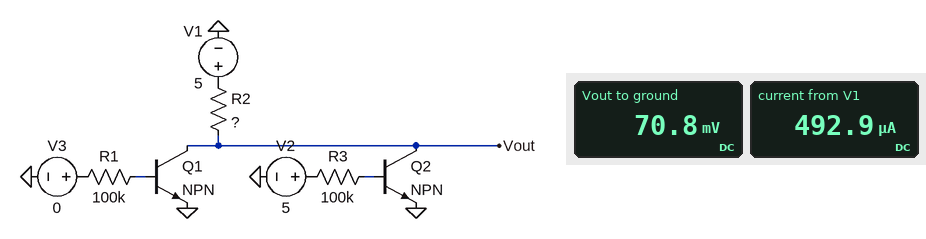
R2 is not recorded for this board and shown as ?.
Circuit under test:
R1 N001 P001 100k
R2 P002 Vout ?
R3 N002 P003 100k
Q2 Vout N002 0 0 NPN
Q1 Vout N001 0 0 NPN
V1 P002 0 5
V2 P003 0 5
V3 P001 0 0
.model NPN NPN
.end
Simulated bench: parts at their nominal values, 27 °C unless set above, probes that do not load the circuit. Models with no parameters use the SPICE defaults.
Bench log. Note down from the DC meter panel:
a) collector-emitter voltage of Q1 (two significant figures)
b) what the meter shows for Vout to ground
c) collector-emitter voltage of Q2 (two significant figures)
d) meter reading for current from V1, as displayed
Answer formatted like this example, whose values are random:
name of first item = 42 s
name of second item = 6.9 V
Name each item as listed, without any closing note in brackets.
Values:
collector-emitter voltage of Q1 = 71 mV
what the meter shows for Vout to ground = 70.8 mV
collector-emitter voltage of Q2 = 71 mV
meter reading for current from V1, as displayed = 492.9 µA
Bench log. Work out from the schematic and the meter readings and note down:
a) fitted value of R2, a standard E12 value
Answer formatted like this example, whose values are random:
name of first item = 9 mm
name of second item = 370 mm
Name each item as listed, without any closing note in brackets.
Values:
fitted value of R2, a standard E12 value = 10 kΩ
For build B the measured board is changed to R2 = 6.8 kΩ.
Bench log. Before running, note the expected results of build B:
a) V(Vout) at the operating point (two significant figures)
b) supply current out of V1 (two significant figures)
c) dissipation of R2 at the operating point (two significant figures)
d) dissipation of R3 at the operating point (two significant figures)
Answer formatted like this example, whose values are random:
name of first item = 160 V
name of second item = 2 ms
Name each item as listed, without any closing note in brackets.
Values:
V(Vout) at the operating point = 81 mV
supply current out of V1 = 720 µA
dissipation of R2 at the operating point = 3.6 mW
dissipation of R3 at the operating point = 180 µW
